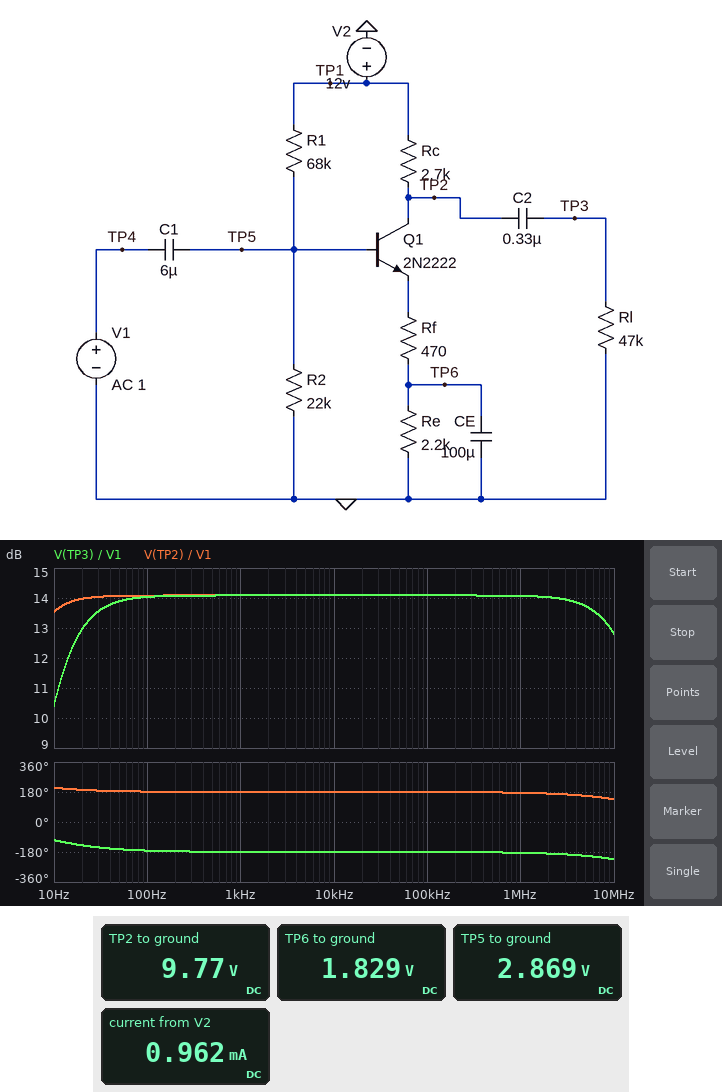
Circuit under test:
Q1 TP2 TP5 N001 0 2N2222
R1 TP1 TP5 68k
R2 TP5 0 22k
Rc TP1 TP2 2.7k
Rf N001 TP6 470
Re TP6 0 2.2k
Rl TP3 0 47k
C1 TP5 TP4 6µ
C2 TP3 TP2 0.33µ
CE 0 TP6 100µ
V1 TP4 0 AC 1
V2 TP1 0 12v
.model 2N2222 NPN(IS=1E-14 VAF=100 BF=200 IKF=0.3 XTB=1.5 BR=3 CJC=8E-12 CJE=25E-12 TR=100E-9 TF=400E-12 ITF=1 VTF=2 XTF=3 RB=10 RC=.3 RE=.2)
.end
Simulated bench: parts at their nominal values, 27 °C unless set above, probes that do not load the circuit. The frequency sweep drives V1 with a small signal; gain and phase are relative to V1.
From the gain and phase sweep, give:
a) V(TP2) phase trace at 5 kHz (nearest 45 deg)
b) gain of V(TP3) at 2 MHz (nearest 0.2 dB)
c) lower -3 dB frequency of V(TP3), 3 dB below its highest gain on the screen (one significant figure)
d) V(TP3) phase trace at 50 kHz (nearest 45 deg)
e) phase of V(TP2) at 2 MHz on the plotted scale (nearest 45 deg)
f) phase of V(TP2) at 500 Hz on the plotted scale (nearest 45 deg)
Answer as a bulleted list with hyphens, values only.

- 180 deg
- 14.0 dB
- 10 Hz
- -180 deg
- 180 deg
- 180 deg
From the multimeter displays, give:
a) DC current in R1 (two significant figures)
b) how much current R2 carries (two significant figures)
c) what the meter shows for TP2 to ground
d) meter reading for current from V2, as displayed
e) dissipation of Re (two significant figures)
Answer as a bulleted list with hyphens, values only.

- 130 µA
- 130 µA
- 9.77 V
- 0.962 mA
- 1.5 mW
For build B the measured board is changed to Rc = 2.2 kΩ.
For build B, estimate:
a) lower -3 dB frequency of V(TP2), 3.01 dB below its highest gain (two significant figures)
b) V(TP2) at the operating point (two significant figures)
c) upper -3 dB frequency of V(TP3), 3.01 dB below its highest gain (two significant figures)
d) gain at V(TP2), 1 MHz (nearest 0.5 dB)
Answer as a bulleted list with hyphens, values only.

- 4.3 Hz
- 10 V
- 23 MHz
- 12.5 dB
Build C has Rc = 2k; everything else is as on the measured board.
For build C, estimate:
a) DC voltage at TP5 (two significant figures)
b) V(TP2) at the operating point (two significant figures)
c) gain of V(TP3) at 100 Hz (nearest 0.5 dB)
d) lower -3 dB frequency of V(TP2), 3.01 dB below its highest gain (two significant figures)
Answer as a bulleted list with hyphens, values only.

- 2.9 V
- 10 V
- 11.5 dB
- 4.3 Hz
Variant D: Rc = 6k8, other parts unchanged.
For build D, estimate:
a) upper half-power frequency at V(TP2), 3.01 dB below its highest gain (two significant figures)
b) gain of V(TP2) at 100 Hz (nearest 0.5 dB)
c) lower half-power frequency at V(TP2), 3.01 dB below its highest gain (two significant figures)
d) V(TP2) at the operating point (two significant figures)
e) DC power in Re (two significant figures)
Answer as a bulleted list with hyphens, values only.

- 5.9 MHz
- 21.5 dB
- 3.8 Hz
- 6.4 V
- 1.5 mW
